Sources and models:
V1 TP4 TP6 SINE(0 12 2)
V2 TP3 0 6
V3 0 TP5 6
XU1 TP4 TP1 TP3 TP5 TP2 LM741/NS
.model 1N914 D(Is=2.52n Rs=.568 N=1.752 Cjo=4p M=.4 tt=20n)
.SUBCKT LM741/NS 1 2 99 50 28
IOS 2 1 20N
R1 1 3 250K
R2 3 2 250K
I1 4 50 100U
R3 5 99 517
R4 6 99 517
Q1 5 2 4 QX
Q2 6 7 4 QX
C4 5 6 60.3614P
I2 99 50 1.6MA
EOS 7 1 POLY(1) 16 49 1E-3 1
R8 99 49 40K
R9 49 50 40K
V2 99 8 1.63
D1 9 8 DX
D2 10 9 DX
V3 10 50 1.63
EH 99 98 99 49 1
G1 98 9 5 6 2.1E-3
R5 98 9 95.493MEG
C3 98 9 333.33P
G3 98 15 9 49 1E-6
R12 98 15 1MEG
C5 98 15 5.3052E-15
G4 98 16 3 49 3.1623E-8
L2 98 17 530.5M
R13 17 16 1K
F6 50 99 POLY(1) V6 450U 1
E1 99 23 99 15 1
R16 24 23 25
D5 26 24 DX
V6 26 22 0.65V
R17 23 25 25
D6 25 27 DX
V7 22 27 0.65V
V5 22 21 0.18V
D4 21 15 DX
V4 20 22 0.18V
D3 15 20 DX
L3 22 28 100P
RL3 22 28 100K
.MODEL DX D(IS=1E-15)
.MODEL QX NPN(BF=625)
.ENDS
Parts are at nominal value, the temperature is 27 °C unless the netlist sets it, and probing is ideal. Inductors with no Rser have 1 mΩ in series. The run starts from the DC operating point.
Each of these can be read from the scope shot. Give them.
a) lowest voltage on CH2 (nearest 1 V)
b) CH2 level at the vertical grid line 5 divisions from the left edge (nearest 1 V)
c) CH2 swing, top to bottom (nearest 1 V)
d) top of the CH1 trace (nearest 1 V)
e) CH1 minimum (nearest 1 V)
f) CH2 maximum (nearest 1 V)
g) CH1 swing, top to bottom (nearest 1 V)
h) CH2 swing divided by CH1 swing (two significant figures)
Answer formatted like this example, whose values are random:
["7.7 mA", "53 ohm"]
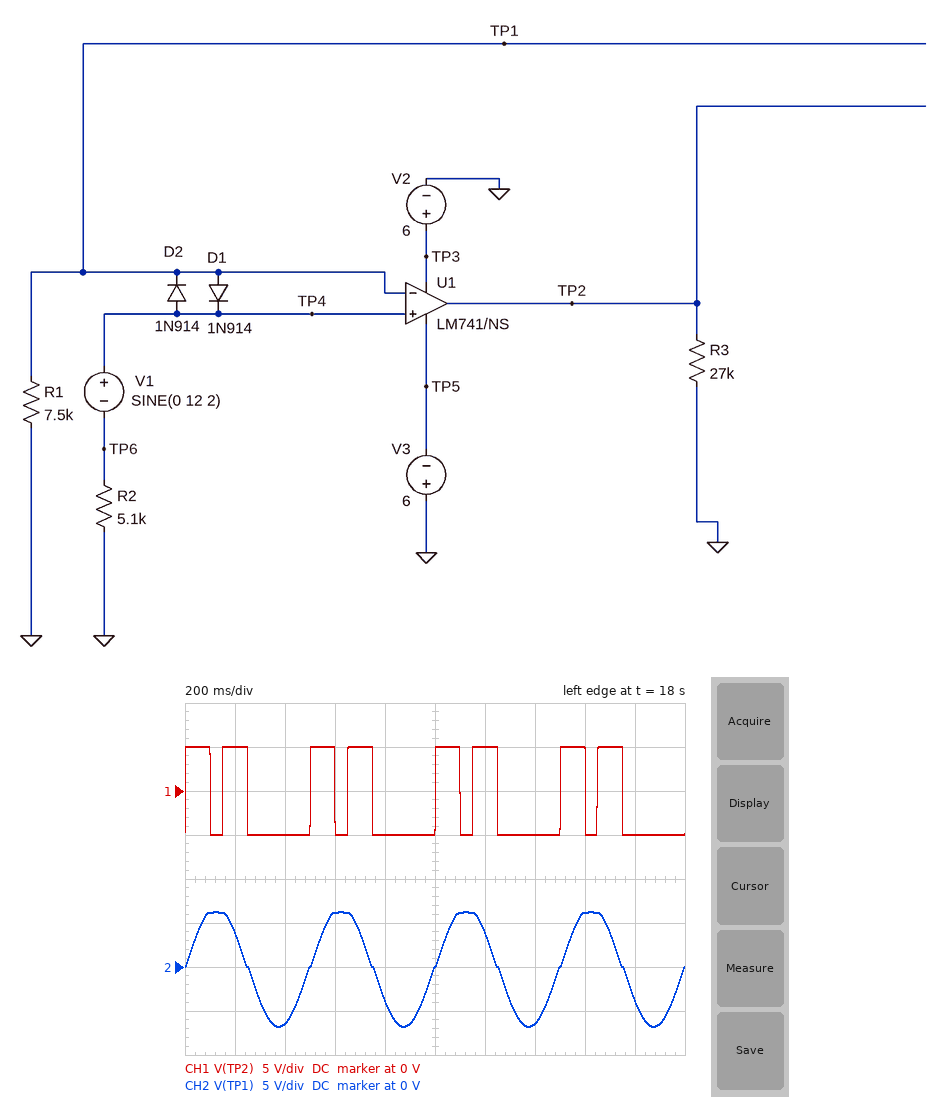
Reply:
["-7 V", "0 V", "13 V", "5 V", "-5 V", "6 V", "10 V", "1.3"]
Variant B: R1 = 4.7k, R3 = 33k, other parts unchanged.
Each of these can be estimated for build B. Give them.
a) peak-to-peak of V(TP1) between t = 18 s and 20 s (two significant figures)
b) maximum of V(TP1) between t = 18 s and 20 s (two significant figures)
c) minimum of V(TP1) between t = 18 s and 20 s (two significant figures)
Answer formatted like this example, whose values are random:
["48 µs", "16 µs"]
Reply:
["11 V", "5.5 V", "-5.5 V"]
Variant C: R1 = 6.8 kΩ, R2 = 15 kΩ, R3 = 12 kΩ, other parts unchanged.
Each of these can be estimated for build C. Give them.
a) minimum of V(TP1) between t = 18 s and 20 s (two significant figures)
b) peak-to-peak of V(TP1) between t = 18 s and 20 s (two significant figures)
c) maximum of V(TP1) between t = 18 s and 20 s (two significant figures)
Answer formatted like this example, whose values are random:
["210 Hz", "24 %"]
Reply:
["-3.6 V", "7.1 V", "3.6 V"]
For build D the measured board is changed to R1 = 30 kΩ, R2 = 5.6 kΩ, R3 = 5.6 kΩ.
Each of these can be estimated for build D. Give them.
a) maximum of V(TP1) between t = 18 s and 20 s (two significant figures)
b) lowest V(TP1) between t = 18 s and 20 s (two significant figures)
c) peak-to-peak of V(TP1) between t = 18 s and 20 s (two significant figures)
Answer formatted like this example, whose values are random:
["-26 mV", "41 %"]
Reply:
["6.5 V", "-9.7 V", "16 V"]
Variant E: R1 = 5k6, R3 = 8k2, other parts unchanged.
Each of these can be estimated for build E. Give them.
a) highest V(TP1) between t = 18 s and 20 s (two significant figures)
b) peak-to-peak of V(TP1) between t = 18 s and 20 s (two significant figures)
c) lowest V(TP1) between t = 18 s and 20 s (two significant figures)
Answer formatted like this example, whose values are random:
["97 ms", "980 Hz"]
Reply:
["6.0 V", "12 V", "-6.0 V"]
